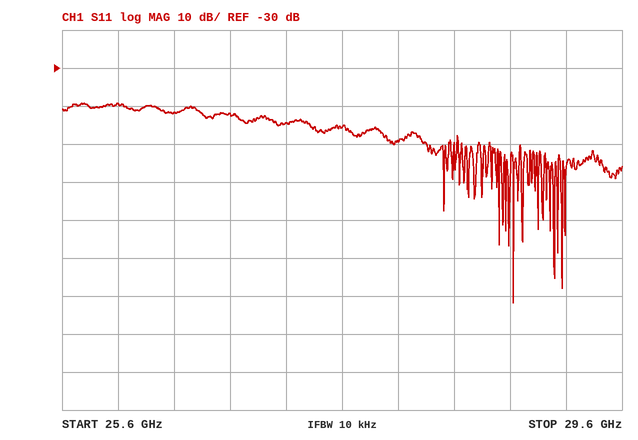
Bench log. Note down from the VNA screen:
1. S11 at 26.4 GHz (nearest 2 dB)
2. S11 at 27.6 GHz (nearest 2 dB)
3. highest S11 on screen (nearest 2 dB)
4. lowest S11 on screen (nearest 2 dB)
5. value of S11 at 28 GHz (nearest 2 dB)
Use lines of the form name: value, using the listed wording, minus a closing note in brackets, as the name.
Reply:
S11 at 26.4 GHz: -42 dB
S11 at 27.6 GHz: -46 dB
highest S11 on screen: -40 dB
lowest S11 on screen: -92 dB
value of S11 at 28 GHz: -50 dB
